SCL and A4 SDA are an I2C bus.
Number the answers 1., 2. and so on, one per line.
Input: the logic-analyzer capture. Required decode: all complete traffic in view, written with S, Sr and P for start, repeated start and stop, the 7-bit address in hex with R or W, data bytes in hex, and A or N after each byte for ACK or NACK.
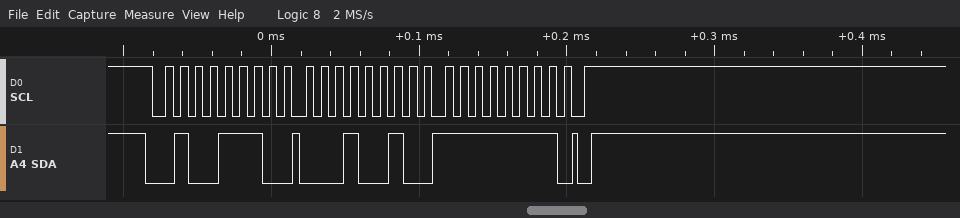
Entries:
1. S 27W A 12 A FF A P
